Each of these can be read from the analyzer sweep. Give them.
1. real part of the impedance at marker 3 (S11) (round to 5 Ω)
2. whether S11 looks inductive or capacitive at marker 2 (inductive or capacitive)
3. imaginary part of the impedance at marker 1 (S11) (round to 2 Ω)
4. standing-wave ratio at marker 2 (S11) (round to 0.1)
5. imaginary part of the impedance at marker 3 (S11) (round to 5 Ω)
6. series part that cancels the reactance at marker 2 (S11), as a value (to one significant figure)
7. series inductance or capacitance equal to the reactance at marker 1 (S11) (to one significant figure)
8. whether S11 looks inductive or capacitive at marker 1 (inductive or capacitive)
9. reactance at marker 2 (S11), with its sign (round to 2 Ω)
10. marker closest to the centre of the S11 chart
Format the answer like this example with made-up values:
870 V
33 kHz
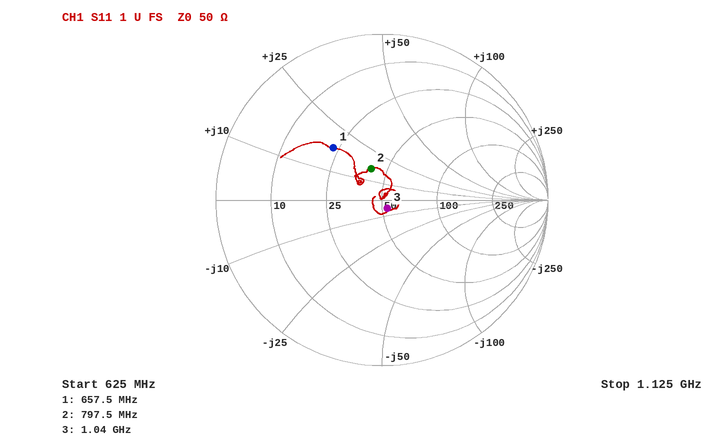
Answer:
55 Ω
inductive
+18 Ω
1.5
-5 Ω
10 pF
4 nH
inductive
+16 Ω
marker 3
